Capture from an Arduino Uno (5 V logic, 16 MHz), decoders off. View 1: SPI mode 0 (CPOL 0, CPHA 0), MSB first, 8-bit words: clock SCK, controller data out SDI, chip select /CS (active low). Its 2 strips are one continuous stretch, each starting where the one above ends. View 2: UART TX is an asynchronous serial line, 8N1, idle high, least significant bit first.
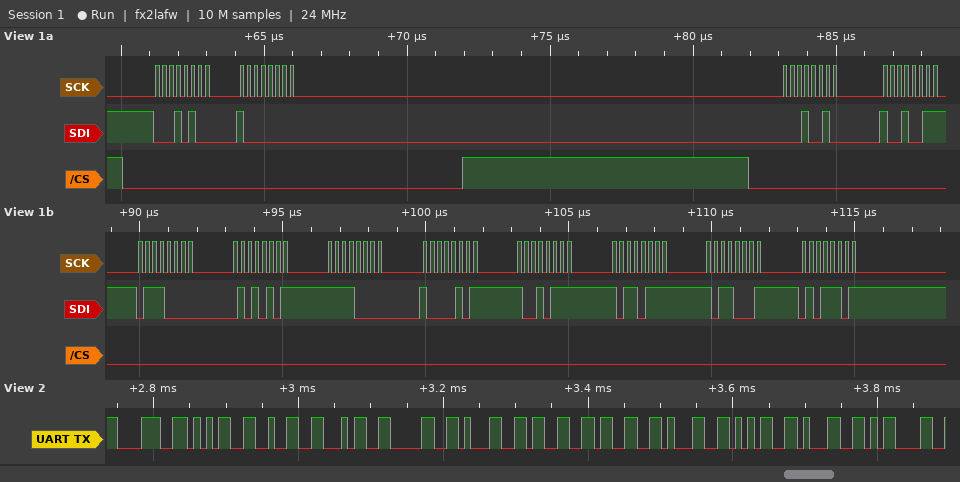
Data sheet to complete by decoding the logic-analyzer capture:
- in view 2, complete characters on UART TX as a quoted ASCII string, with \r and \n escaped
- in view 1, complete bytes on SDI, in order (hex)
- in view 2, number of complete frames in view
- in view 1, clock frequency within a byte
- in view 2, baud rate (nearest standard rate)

"85240133151\r"
0x14 0x80 0x12 0x93 0x70 0x55 0xF0 0x85 0x97 0xB7 0xB1 0x5D
12
4 MHz
115200 baud
